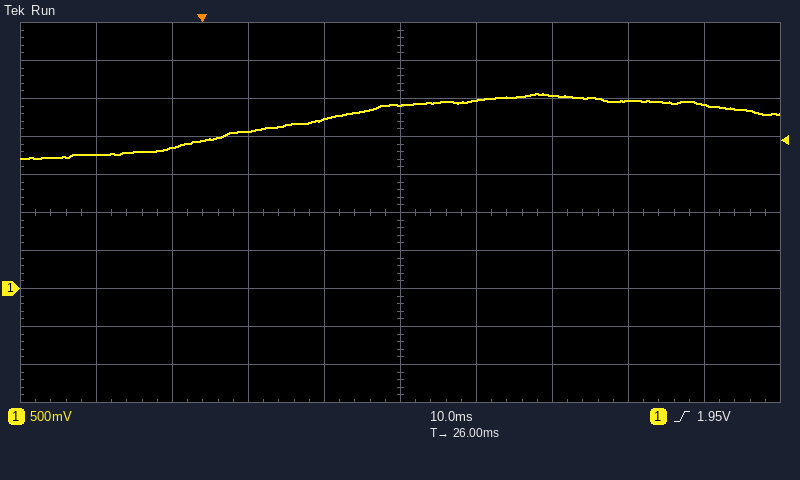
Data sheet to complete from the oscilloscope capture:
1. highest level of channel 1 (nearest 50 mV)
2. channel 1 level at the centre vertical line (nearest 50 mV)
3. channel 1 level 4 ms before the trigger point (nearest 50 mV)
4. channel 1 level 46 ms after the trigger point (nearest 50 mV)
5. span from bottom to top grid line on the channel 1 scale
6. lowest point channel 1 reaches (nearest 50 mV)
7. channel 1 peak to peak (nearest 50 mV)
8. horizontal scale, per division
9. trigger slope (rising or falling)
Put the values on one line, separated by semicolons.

2.55 V; 2.40 V; 1.85 V; 2.55 V; 5 V; 1.70 V; 850 mV; 10 ms; rising
